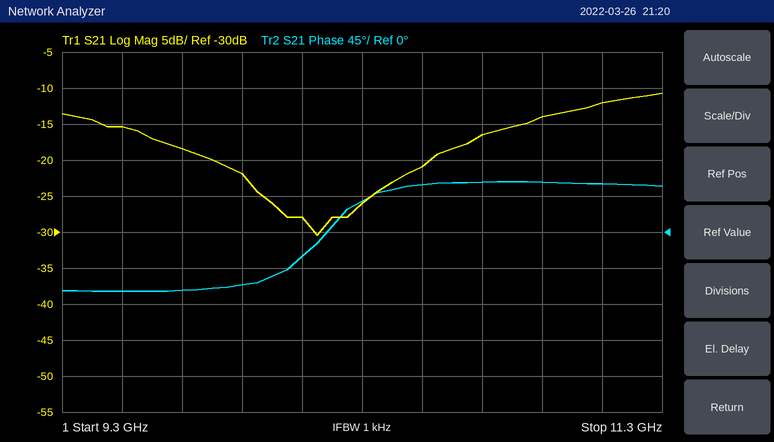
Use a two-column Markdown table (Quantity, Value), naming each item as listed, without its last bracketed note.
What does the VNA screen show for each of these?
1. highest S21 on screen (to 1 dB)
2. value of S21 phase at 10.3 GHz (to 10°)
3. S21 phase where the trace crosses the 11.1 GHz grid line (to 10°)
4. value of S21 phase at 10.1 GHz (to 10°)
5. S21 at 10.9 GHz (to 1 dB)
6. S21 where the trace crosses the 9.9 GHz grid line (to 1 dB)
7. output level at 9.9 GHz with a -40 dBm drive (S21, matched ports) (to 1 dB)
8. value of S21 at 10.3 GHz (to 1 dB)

| Quantity | Value |
|---|---|
| highest S21 on screen | -11 dB |
| value of S21 phase at 10.3 GHz | 40° |
| S21 phase where the trace crosses the 11.1 GHz grid line | 60° |
| value of S21 phase at 10.1 GHz | -30° |
| S21 at 10.9 GHz | -14 dB |
| S21 where the trace crosses the 9.9 GHz grid line | -22 dB |
| output level at 9.9 GHz with a -40 dBm drive (S21, matched ports) | -62 dBm |
| value of S21 at 10.3 GHz | -26 dB |
